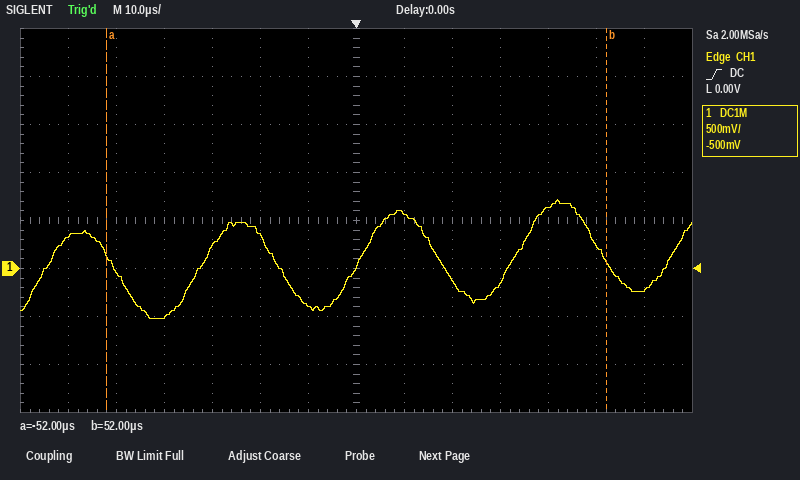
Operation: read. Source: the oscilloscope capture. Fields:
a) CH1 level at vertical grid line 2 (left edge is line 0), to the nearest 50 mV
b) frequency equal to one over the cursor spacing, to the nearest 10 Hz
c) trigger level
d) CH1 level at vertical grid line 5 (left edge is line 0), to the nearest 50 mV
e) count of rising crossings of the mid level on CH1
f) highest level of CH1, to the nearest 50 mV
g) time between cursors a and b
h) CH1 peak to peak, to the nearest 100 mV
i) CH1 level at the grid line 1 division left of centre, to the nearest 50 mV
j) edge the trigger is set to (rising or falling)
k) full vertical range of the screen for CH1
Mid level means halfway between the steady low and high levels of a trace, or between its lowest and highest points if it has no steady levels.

-50 mV
9.62 kHz
0.00 V
350 mV
5
700 mV
104 µs
1.20 V
-400 mV
rising
4 V
